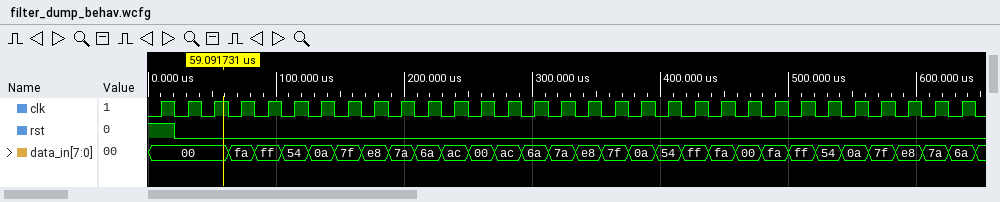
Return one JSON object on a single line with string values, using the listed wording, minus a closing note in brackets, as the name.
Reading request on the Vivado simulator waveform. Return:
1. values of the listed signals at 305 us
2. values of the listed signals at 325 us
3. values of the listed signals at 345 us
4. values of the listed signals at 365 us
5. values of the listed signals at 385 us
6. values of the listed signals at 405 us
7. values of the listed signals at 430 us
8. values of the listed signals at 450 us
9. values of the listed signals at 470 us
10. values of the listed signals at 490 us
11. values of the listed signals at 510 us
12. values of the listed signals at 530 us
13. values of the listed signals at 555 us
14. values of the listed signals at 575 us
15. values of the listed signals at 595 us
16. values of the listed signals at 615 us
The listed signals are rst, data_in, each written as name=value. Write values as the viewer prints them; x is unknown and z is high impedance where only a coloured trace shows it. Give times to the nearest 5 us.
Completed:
{"values of the listed signals at 305 us": "rst=0, data_in=6a", "values of the listed signals at 325 us": "rst=0, data_in=7a", "values of the listed signals at 345 us": "rst=0, data_in=e8", "values of the listed signals at 365 us": "rst=0, data_in=7f", "values of the listed signals at 385 us": "rst=0, data_in=0a", "values of the listed signals at 405 us": "rst=0, data_in=54", "values of the listed signals at 430 us": "rst=0, data_in=ff", "values of the listed signals at 450 us": "rst=0, data_in=fa", "values of the listed signals at 470 us": "rst=0, data_in=00", "values of the listed signals at 490 us": "rst=0, data_in=fa", "values of the listed signals at 510 us": "rst=0, data_in=ff", "values of the listed signals at 530 us": "rst=0, data_in=54", "values of the listed signals at 555 us": "rst=0, data_in=0a", "values of the listed signals at 575 us": "rst=0, data_in=7f", "values of the listed signals at 595 us": "rst=0, data_in=e8", "values of the listed signals at 615 us": "rst=0, data_in=7a"}
